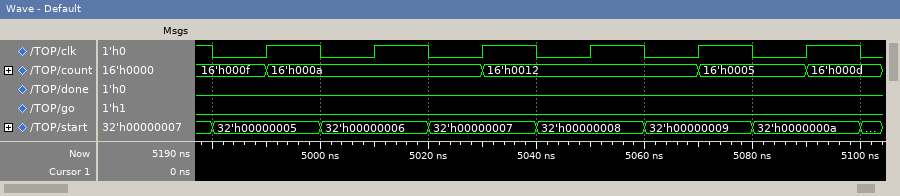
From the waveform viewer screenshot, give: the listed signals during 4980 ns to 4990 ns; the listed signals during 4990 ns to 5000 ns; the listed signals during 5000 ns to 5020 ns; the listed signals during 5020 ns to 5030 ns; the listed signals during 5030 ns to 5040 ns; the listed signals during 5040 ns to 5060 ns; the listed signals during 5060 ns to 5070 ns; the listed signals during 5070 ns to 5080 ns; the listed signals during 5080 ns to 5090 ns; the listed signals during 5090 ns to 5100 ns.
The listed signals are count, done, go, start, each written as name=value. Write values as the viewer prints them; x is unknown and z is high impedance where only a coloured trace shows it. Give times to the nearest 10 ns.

count=16'h000f, done=0, go=0, start=32'h00000005
count=16'h000a, done=0, go=0, start=32'h00000005
count=16'h000a, done=0, go=0, start=32'h00000006
count=16'h000a, done=0, go=0, start=32'h00000007
count=16'h0012, done=0, go=0, start=32'h00000007
count=16'h0012, done=0, go=0, start=32'h00000008
count=16'h0012, done=0, go=0, start=32'h00000009
count=16'h0005, done=0, go=0, start=32'h00000009
count=16'h0005, done=0, go=0, start=32'h0000000a
count=16'h000d, done=0, go=0, start=32'h0000000a
